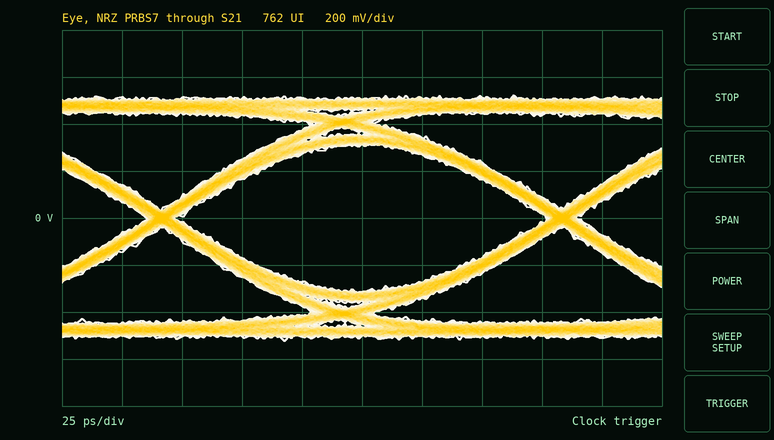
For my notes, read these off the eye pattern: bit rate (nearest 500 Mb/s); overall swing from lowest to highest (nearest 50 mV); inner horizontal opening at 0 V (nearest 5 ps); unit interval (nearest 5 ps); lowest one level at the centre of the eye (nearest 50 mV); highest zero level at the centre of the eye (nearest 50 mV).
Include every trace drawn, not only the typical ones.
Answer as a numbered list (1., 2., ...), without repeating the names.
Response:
1. 6.0 Gb/s
2. 1.05 V
3. 155 ps
4. 165 ps
5. 300 mV
6. -300 mV
